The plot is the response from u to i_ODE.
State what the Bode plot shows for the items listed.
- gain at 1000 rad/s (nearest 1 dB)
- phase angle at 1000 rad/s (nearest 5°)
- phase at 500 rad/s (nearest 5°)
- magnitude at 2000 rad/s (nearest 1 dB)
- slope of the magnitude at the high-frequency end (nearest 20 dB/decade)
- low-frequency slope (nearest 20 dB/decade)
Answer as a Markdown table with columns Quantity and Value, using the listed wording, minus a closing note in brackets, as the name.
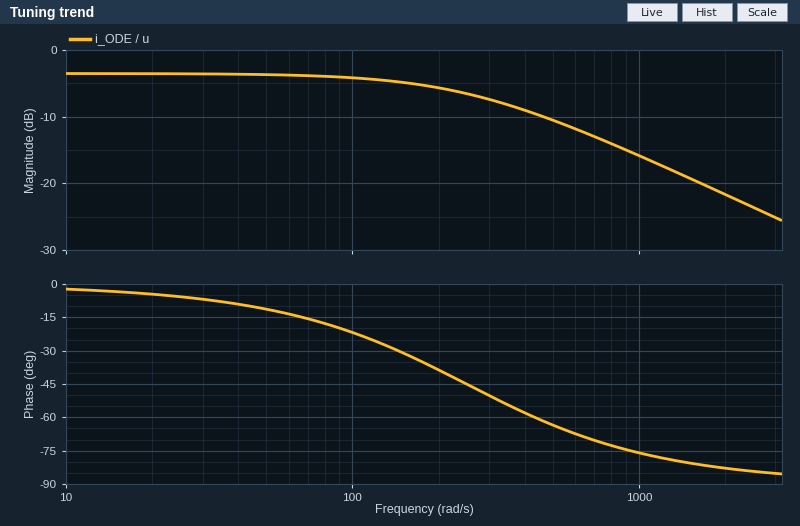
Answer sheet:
| Quantity | Value |
|---|---|
| gain at 1000 rad/s | -16 dB |
| phase angle at 1000 rad/s | -75° |
| phase at 500 rad/s | -65° |
| magnitude at 2000 rad/s | -22 dB |
| slope of the magnitude at the high-frequency end | -20 dB/decade |
| low-frequency slope | 0 dB/decade |
